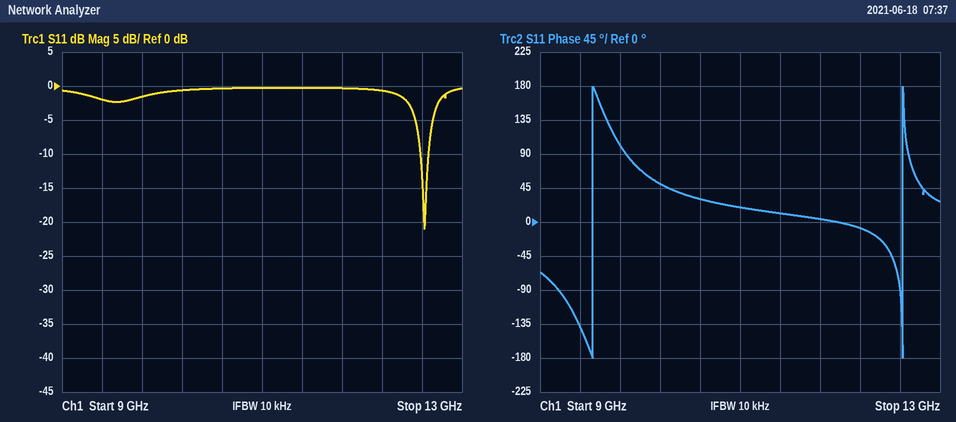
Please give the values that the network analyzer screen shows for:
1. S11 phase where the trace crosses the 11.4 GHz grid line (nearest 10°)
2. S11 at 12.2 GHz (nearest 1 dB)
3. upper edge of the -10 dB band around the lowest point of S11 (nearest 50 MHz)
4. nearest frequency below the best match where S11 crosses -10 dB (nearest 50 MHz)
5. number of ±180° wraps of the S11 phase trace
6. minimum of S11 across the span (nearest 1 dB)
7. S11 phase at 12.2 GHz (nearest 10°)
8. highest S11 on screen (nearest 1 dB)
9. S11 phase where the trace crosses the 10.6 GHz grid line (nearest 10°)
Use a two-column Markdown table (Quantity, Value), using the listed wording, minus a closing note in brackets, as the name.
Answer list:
| Quantity | Value |
|---|---|
| S11 phase where the trace crosses the 11.4 GHz grid line | 10° |
| S11 at 12.2 GHz | -1 dB |
| upper edge of the -10 dB band around the lowest point of S11 | 12.65 GHz |
| nearest frequency below the best match where S11 crosses -10 dB | 12.60 GHz |
| number of ±180° wraps of the S11 phase trace | 2 |
| minimum of S11 across the span | -21 dB |
| S11 phase at 12.2 GHz | -10° |
| highest S11 on screen | 0 dB |
| S11 phase where the trace crosses the 10.6 GHz grid line | 30° |
